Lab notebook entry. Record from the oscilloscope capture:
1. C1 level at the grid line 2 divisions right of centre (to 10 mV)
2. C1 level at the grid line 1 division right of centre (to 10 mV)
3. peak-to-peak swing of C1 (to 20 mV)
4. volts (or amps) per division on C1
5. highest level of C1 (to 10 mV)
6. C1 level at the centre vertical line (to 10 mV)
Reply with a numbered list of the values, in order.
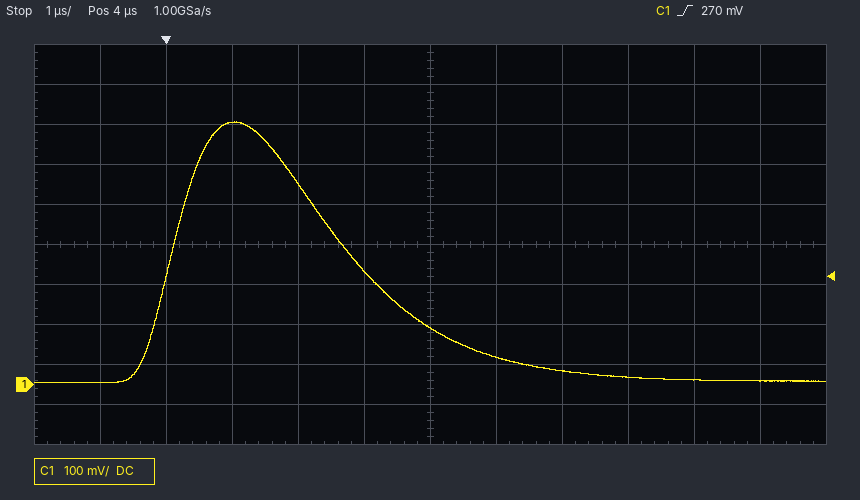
1. 30 mV
2. 70 mV
3. 660 mV
4. 100 mV
5. 660 mV
6. 140 mV
